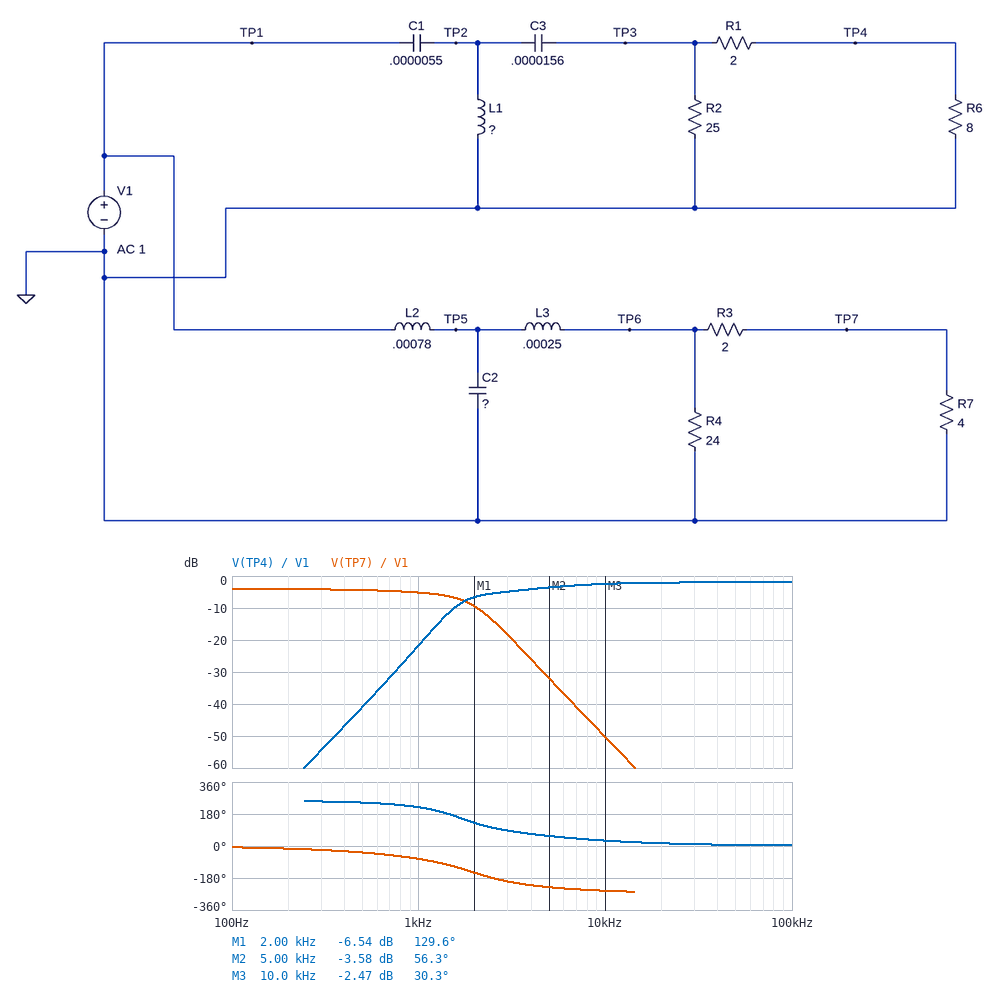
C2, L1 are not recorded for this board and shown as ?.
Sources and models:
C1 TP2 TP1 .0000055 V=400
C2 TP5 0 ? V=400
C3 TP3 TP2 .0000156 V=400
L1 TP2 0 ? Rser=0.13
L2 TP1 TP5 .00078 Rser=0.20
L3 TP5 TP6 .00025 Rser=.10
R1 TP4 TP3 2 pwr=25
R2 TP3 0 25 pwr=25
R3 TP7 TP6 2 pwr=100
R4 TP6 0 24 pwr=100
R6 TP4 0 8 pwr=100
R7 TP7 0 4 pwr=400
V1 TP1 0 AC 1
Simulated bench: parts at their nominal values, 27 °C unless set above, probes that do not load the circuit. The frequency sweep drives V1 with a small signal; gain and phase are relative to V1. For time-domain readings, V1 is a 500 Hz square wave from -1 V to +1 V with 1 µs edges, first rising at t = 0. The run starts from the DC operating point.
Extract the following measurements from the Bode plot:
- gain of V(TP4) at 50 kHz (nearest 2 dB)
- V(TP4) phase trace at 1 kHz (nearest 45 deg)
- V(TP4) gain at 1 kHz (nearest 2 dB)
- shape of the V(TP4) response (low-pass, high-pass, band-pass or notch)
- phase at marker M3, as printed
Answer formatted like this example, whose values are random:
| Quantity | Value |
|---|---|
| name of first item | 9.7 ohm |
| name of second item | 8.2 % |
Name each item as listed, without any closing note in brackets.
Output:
| Quantity | Value |
|---|---|
| gain of V(TP4) at 50 kHz | -2 dB |
| V(TP4) phase trace at 1 kHz | 225 deg |
| V(TP4) gain at 1 kHz | -22 dB |
| shape of the V(TP4) response | high-pass |
| phase at marker M3, as printed | 30.3 deg |
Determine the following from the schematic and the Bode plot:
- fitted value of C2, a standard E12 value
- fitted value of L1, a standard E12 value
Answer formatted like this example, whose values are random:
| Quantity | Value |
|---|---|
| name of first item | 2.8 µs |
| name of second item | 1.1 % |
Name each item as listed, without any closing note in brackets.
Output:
| Quantity | Value |
|---|---|
| fitted value of C2, a standard E12 value | 22 µF |
| fitted value of L1, a standard E12 value | 560 µH |
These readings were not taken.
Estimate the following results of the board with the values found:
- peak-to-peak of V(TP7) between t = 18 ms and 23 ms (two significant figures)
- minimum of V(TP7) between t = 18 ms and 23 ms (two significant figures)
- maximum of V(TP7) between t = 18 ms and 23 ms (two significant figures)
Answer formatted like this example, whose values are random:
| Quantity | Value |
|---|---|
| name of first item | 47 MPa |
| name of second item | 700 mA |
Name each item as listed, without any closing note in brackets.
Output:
| Quantity | Value |
|---|---|
| peak-to-peak of V(TP7) between t = 18 ms and 23 ms | 1.3 V |
| minimum of V(TP7) between t = 18 ms and 23 ms | -650 mV |
| maximum of V(TP7) between t = 18 ms and 23 ms | 650 mV |
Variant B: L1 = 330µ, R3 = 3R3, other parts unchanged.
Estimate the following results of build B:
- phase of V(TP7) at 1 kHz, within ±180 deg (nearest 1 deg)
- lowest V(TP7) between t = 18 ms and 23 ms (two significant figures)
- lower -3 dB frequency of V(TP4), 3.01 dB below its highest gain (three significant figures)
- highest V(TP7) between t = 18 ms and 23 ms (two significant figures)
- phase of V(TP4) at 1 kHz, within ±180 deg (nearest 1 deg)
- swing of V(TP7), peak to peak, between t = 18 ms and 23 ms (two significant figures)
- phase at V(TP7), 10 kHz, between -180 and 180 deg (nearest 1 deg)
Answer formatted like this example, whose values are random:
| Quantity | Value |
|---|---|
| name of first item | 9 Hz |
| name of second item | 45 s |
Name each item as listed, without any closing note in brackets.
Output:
| Quantity | Value |
|---|---|
| phase of V(TP7) at 1 kHz, within ±180 deg | -70 deg |
| lowest V(TP7) between t = 18 ms and 23 ms | -610 mV |
| lower -3 dB frequency of V(TP4), 3.01 dB below its highest gain | 2.70 kHz |
| highest V(TP7) between t = 18 ms and 23 ms | 610 mV |
| phase of V(TP4) at 1 kHz, within ±180 deg | -136 deg |
| swing of V(TP7), peak to peak, between t = 18 ms and 23 ms | 1.2 V |
| phase at V(TP7), 10 kHz, between -180 and 180 deg | 111 deg |
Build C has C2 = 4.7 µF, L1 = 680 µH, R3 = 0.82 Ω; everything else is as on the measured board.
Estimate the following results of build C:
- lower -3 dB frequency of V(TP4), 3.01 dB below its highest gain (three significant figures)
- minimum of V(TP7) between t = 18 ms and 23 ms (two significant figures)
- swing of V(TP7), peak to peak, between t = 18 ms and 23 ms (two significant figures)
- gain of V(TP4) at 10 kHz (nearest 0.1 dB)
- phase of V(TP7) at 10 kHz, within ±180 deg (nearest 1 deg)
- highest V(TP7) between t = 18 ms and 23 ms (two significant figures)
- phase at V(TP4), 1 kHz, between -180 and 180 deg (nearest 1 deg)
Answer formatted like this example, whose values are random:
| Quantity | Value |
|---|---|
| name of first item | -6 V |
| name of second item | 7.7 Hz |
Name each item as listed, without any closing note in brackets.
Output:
| Quantity | Value |
|---|---|
| lower -3 dB frequency of V(TP4), 3.01 dB below its highest gain | 3.52 kHz |
| minimum of V(TP7) between t = 18 ms and 23 ms | -750 mV |
| swing of V(TP7), peak to peak, between t = 18 ms and 23 ms | 1.5 V |
| gain of V(TP4) at 10 kHz | -2.6 dB |
| phase of V(TP7) at 10 kHz, within ±180 deg | 109 deg |
| highest V(TP7) between t = 18 ms and 23 ms | 750 mV |
| phase at V(TP4), 1 kHz, between -180 and 180 deg | -147 deg |
